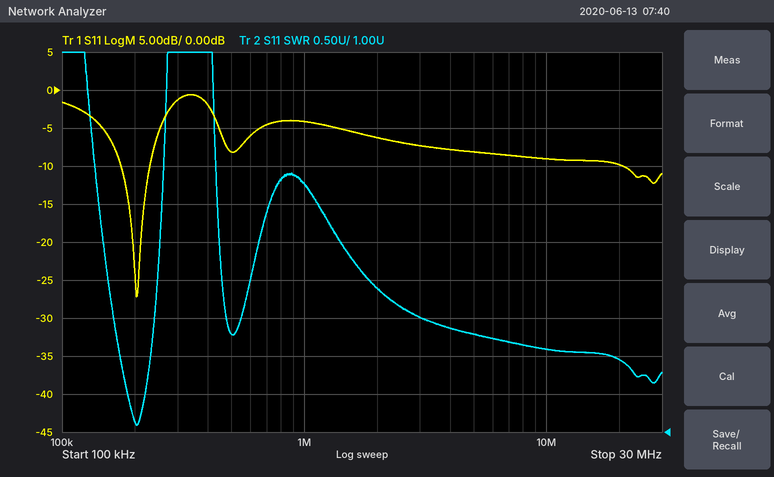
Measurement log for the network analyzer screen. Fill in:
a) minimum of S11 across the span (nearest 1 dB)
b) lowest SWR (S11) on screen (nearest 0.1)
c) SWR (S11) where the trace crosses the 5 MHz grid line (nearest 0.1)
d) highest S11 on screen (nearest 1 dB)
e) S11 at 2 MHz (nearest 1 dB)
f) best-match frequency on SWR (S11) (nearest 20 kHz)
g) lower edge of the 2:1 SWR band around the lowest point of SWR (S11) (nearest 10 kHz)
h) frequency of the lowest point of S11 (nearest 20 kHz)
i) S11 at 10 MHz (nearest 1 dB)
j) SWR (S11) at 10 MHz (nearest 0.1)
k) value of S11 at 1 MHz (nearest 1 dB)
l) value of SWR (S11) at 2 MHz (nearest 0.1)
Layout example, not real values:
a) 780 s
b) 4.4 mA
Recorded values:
a) -27 dB
b) 1.1
c) 2.3
d) -1 dB
e) -6 dB
f) 200 kHz
g) 170 kHz
h) 200 kHz
i) -9 dB
j) 2.1
k) -4 dB
l) 2.9
